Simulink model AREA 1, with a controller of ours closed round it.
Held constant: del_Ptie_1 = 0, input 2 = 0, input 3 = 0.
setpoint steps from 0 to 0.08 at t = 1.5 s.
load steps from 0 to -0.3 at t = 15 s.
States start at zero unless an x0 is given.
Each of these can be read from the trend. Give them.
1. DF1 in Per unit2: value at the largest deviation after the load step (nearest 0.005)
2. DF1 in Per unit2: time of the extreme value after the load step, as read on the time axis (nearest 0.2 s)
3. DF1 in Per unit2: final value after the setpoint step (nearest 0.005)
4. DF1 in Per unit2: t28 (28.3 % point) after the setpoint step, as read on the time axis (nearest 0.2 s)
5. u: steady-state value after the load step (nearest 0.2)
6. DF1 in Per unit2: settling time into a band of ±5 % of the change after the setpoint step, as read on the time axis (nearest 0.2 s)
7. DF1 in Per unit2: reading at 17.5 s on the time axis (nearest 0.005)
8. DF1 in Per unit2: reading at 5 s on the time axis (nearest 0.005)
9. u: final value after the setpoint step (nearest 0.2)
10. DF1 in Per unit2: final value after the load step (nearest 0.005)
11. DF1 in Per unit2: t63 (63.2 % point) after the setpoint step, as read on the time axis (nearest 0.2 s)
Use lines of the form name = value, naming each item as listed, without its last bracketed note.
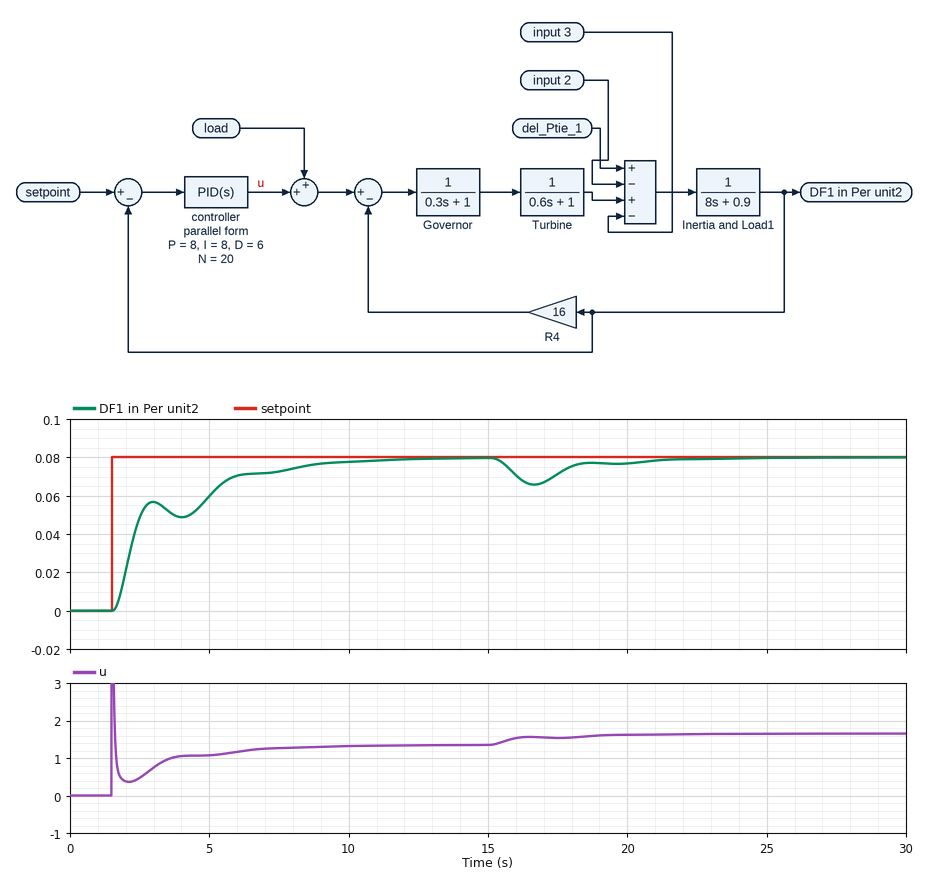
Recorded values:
DF1 in Per unit2: value at the largest deviation after the load step = 0.065
DF1 in Per unit2: time of the extreme value after the load step, as read on the time axis = 16.6 s
DF1 in Per unit2: final value after the setpoint step = 0.080
DF1 in Per unit2: t28 (28.3 % point) after the setpoint step, as read on the time axis = 2.0 s
u: steady-state value after the load step = 1.6
DF1 in Per unit2: settling time into a band of ±5 % of the change after the setpoint step, as read on the time axis = 8.6 s
DF1 in Per unit2: reading at 17.5 s on the time axis = 0.070
DF1 in Per unit2: reading at 5 s on the time axis = 0.060
u: final value after the setpoint step = 1.4
DF1 in Per unit2: final value after the load step = 0.080
DF1 in Per unit2: t63 (63.2 % point) after the setpoint step, as read on the time axis = 2.6 s
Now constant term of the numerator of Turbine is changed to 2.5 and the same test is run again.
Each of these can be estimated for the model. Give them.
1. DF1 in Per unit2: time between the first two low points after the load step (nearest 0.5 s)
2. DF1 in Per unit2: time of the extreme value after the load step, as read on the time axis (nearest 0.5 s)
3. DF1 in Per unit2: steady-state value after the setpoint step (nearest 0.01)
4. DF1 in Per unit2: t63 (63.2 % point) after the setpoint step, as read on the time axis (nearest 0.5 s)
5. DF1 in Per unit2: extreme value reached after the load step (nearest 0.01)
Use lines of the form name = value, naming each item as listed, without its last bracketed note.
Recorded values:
DF1 in Per unit2: time between the first two low points after the load step = 2.0 s
DF1 in Per unit2: time of the extreme value after the load step, as read on the time axis = 16.0 s
DF1 in Per unit2: steady-state value after the setpoint step = 0.08
DF1 in Per unit2: t63 (63.2 % point) after the setpoint step, as read on the time axis = 2.0 s
DF1 in Per unit2: extreme value reached after the load step = 0.06
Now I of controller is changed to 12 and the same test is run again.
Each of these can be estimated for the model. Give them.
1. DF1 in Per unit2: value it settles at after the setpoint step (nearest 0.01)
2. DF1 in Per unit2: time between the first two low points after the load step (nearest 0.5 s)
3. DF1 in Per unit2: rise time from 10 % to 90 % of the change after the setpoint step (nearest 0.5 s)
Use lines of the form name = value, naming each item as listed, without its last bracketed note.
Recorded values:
DF1 in Per unit2: value it settles at after the setpoint step = 0.08
DF1 in Per unit2: time between the first two low points after the load step = 3.5 s
DF1 in Per unit2: rise time from 10 % to 90 % of the change after the setpoint step = 3.5 s
